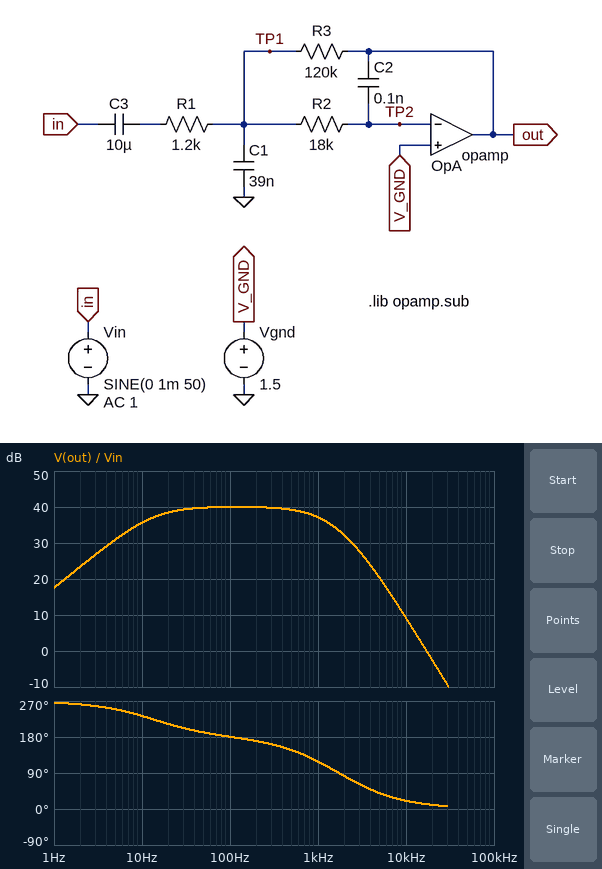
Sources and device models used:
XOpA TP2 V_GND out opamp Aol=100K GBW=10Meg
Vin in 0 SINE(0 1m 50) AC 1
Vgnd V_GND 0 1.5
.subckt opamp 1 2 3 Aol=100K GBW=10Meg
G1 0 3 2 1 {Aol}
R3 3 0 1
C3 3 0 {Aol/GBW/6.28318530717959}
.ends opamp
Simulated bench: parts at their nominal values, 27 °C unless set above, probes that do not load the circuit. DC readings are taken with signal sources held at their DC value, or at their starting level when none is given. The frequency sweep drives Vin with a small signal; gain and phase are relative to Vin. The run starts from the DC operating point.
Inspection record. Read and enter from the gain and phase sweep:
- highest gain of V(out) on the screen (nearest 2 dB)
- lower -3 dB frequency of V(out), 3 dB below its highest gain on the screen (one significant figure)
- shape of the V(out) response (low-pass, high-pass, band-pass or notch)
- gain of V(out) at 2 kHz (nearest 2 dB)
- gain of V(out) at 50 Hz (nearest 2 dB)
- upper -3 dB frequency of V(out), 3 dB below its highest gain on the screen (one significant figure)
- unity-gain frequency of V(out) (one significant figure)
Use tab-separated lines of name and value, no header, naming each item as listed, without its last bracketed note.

highest gain of V(out) on the screen	40 dB
lower -3 dB frequency of V(out), 3 dB below its highest gain on the screen	10 Hz
shape of the V(out) response	band-pass
gain of V(out) at 2 kHz	32 dB
gain of V(out) at 50 Hz	40 dB
upper -3 dB frequency of V(out), 3 dB below its highest gain on the screen	1 kHz
unity-gain frequency of V(out)	20 kHz
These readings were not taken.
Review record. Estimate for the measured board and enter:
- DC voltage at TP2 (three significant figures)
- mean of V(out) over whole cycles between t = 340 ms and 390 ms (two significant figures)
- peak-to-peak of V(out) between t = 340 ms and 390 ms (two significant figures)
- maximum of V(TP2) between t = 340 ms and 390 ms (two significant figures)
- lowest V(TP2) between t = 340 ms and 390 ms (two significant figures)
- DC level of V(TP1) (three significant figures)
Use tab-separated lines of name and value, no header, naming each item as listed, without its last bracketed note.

DC voltage at TP2	1.50 V
mean of V(out) over whole cycles between t = 340 ms and 390 ms	1.5 V
peak-to-peak of V(out) between t = 340 ms and 390 ms	200 mV
maximum of V(TP2) between t = 340 ms and 390 ms	1.5 V
lowest V(TP2) between t = 340 ms and 390 ms	1.5 V
DC level of V(TP1)	1.50 V
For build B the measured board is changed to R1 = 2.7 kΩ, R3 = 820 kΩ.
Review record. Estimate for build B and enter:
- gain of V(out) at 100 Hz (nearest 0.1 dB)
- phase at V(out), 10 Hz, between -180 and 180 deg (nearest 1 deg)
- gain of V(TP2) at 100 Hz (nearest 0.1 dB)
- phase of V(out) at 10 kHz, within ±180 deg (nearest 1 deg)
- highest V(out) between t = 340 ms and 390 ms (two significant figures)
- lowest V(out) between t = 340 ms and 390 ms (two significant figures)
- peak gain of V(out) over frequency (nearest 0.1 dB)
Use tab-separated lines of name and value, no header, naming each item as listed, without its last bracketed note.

gain of V(out) at 100 Hz	49.3 dB
phase at V(out), 10 Hz, between -180 and 180 deg	-151 deg
gain of V(TP2) at 100 Hz	-47.7 dB
phase of V(out) at 10 kHz, within ±180 deg	10 deg
highest V(out) between t = 340 ms and 390 ms	1.8 V
lowest V(out) between t = 340 ms and 390 ms	1.2 V
peak gain of V(out) over frequency	49.6 dB
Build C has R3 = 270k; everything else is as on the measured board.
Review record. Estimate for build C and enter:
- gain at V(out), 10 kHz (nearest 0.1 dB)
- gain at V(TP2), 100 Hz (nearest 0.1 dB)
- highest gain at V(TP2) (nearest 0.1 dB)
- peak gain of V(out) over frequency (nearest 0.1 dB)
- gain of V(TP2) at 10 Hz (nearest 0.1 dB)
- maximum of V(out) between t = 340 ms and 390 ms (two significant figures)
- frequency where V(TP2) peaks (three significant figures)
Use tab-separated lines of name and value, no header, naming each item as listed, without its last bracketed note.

gain at V(out), 10 kHz	9.0 dB
gain at V(TP2), 100 Hz	-50.0 dB
highest gain at V(TP2)	-41.7 dB
peak gain of V(out) over frequency	47.0 dB
gain of V(TP2) at 10 Hz	-57.2 dB
maximum of V(out) between t = 340 ms and 390 ms	1.7 V
frequency where V(TP2) peaks	1.11 kHz
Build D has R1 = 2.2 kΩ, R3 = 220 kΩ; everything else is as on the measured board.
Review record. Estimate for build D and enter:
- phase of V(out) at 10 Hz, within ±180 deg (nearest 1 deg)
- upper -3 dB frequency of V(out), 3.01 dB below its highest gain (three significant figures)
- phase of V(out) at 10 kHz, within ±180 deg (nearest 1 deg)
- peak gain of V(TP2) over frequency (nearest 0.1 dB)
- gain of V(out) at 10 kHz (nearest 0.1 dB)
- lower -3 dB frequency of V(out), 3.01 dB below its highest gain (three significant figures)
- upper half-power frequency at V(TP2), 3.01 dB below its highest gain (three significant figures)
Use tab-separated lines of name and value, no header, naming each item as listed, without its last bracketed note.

phase of V(out) at 10 Hz, within ±180 deg	-145 deg
upper -3 dB frequency of V(out), 3.01 dB below its highest gain	1.07 kHz
phase of V(out) at 10 kHz, within ±180 deg	12 deg
peak gain of V(TP2) over frequency	-42.2 dB
gain of V(out) at 10 kHz	4.2 dB
lower -3 dB frequency of V(out), 3.01 dB below its highest gain	7.22 Hz
upper half-power frequency at V(TP2), 3.01 dB below its highest gain	2.69 kHz
